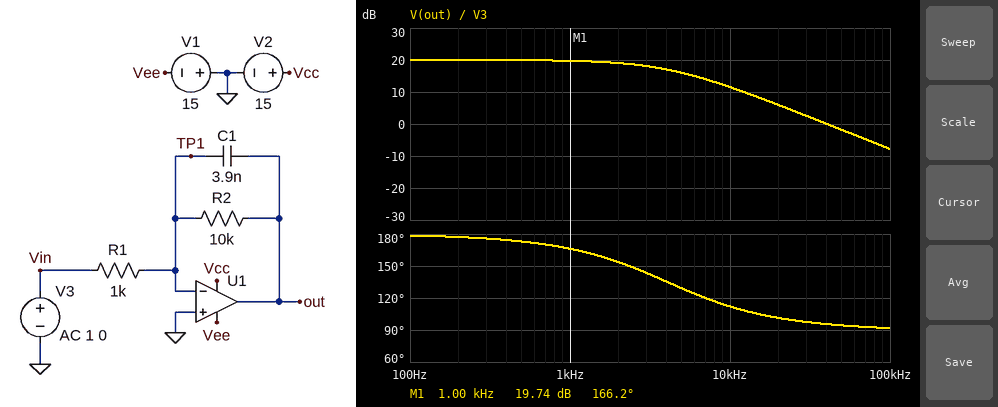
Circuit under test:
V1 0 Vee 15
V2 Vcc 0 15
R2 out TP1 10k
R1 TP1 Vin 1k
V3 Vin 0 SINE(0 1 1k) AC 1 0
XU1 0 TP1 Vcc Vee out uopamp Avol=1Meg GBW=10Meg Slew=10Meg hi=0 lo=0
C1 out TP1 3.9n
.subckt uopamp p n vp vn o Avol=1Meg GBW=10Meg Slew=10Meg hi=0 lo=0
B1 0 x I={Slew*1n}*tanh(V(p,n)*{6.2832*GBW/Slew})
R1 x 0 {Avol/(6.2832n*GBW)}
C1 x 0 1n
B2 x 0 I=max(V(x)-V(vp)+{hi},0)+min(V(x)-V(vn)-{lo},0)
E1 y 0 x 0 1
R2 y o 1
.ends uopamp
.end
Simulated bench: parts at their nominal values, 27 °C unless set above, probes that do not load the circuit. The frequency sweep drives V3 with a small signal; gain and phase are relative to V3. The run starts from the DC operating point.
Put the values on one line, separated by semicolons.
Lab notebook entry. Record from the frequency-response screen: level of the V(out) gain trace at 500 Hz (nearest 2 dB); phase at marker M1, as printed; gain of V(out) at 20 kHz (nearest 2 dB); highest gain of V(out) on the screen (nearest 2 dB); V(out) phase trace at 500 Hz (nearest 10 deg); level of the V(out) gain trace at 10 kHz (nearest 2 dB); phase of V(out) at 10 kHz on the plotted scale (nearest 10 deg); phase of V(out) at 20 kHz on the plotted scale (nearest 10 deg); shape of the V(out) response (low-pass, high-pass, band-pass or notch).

20 dB; 166.2 deg; 6 dB; 20 dB; 170 deg; 12 dB; 110 deg; 100 deg; low-pass
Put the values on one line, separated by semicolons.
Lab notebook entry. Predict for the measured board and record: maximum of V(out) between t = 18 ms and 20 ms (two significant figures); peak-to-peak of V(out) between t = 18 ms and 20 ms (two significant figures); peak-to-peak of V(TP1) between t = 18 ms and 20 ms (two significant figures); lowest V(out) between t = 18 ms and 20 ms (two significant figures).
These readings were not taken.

9.7 V; 19 V; 1.9 mV; -9.7 V
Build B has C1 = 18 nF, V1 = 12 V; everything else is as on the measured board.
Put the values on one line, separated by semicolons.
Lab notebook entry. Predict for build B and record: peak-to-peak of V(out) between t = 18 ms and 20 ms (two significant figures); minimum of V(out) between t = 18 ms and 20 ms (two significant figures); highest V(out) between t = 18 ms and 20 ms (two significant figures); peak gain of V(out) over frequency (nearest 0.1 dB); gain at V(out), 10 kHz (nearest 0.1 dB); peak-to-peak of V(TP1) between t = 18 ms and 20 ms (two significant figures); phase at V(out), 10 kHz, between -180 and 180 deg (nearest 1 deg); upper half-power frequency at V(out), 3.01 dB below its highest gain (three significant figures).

13 V; -6.6 V; 6.6 V; 20.0 dB; -1.1 dB; 1.3 mV; 95 deg; 883 Hz
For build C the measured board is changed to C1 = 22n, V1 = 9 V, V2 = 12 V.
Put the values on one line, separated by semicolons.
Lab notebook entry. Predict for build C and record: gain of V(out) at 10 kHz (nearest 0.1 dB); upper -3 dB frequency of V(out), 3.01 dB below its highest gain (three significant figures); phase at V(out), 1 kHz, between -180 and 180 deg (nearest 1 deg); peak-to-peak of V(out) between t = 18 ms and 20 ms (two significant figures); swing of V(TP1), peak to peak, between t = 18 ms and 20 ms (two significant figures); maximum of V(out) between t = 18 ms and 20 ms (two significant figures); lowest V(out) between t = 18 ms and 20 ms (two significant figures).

-2.8 dB; 723 Hz; 126 deg; 12 V; 1.2 mV; 5.9 V; -5.9 V
